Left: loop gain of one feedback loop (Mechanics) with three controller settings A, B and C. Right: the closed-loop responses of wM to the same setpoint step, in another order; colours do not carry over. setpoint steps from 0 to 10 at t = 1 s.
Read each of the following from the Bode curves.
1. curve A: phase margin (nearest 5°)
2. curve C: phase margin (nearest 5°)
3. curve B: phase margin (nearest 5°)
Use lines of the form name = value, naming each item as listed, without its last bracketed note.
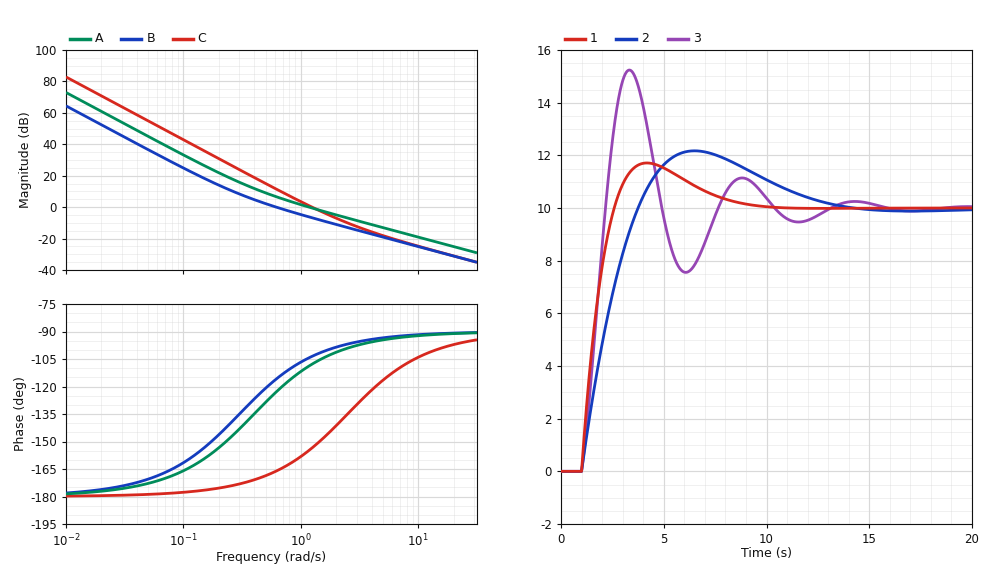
curve A: phase margin = 70°
curve C: phase margin = 25°
curve B: phase margin = 65°
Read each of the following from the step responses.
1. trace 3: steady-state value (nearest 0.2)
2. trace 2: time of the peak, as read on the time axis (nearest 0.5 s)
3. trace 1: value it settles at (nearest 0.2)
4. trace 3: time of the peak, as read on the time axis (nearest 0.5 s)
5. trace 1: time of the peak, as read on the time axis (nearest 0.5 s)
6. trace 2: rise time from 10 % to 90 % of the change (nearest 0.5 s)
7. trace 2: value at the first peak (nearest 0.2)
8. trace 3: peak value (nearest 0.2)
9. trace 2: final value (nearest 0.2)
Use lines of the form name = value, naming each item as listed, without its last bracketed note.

trace 3: steady-state value = 10.0
trace 2: time of the peak, as read on the time axis = 6.5 s
trace 1: value it settles at = 10.0
trace 3: time of the peak, as read on the time axis = 3.5 s
trace 1: time of the peak, as read on the time axis = 4.0 s
trace 2: rise time from 10 % to 90 % of the change = 2.0 s
trace 2: value at the first peak = 12.2
trace 3: peak value = 15.2
trace 2: final value = 10.0
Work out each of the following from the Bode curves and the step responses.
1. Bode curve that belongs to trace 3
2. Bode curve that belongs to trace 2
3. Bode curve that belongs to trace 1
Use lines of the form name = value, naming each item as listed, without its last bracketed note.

Bode curve that belongs to trace 3 = C
Bode curve that belongs to trace 2 = B
Bode curve that belongs to trace 1 = A
